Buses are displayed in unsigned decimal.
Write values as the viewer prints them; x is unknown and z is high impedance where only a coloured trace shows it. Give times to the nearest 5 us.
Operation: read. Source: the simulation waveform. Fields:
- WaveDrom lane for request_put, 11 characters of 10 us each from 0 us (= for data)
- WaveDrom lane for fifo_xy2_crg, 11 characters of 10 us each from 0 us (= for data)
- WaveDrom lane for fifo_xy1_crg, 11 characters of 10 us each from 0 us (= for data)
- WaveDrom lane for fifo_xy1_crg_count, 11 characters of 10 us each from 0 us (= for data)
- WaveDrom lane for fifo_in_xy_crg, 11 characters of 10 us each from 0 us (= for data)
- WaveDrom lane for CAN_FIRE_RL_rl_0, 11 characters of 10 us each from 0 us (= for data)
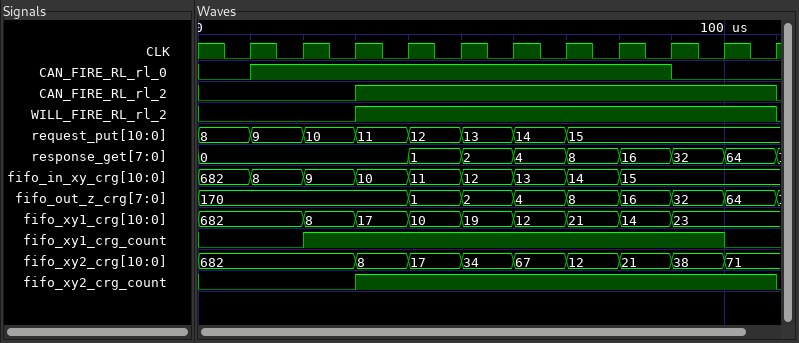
{name: 'request_put', wave: '========...', data: '8 9 10 11 12 13 14 15'}
{name: 'fifo_xy2_crg', wave: '=..========', data: '682 8 17 34 67 12 21 38 71'}
{name: 'fifo_xy1_crg', wave: '=.========.', data: '682 8 17 10 19 12 21 14 23'}
{name: 'fifo_xy1_crg_count', wave: '0.1.......0'}
{name: 'fifo_in_xy_crg', wave: '=========..', data: '682 8 9 10 11 12 13 14 15'}
{name: 'CAN_FIRE_RL_rl_0', wave: '01.......0.'}
